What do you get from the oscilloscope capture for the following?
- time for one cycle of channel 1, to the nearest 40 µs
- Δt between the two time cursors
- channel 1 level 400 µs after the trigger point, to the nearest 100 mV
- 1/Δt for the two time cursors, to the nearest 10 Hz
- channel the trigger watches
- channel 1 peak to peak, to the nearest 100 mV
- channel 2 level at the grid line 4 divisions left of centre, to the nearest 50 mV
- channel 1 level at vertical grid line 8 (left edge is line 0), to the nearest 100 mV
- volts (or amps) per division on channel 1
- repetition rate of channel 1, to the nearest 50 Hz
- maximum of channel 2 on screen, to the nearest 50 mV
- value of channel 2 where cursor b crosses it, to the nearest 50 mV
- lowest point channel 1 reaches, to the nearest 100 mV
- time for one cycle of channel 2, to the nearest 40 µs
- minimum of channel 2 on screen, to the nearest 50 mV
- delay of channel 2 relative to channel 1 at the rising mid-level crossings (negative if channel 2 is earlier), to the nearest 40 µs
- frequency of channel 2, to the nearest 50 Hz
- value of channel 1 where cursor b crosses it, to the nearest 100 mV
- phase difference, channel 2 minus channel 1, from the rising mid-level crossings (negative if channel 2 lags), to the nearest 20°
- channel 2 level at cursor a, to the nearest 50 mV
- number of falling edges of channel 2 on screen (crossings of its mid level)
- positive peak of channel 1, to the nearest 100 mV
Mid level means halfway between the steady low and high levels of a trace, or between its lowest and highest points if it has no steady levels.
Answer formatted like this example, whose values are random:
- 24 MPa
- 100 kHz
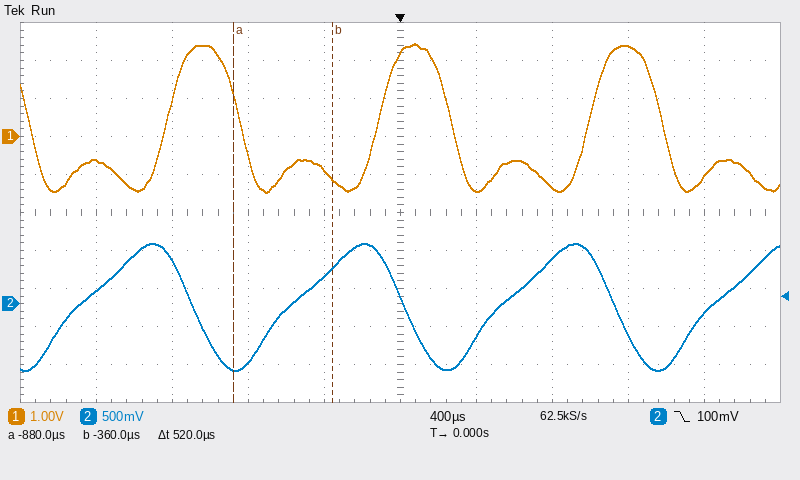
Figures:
- 1.12 ms
- 520 µs
- -1.4 V
- 1.92 kHz
- channel 2
- 3.9 V
- 150 mV
- 2.4 V
- 1 V
- 900 Hz
- 800 mV
- 450 mV
- -1.5 V
- 1.12 ms
- -900 mV
- -480 µs
- 900 Hz
- -1.1 V
- +160°
- -850 mV
- 3
- 2.4 V
